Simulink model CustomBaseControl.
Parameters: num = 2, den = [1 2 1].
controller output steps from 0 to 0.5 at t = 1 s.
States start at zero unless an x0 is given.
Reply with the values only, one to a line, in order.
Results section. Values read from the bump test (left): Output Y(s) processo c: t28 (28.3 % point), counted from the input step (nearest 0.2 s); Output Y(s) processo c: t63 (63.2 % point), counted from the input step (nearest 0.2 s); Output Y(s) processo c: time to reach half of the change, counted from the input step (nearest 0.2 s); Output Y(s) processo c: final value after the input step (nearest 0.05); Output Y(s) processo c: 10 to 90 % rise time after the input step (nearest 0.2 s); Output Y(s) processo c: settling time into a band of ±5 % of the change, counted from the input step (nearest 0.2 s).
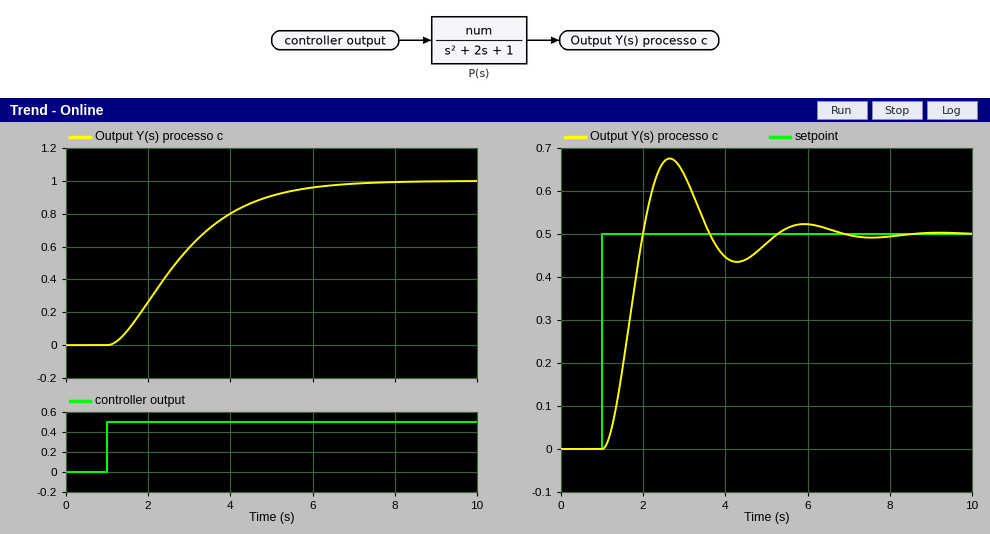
1.0 s
2.2 s
1.6 s
1.00
3.4 s
4.8 s
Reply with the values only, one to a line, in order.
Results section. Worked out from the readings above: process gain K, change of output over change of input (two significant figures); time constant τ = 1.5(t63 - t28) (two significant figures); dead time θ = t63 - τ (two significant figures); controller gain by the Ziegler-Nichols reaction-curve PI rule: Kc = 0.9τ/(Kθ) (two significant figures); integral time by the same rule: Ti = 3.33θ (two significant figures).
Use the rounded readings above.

2.0
1.8 s
0.40 s
2.0
1.3 s
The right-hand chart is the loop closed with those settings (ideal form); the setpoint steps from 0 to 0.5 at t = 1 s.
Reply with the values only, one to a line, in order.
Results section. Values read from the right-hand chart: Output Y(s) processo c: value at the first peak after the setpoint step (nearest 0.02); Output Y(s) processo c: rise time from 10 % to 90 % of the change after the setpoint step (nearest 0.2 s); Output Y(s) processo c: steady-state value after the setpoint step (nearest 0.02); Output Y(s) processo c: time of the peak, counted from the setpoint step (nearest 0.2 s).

0.68
0.6 s
0.50
1.6 s
